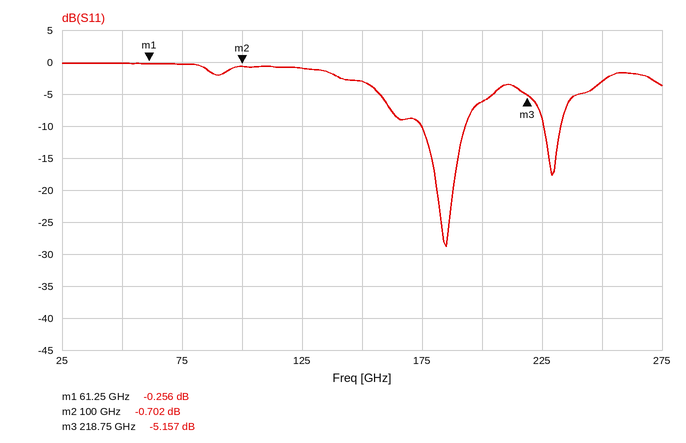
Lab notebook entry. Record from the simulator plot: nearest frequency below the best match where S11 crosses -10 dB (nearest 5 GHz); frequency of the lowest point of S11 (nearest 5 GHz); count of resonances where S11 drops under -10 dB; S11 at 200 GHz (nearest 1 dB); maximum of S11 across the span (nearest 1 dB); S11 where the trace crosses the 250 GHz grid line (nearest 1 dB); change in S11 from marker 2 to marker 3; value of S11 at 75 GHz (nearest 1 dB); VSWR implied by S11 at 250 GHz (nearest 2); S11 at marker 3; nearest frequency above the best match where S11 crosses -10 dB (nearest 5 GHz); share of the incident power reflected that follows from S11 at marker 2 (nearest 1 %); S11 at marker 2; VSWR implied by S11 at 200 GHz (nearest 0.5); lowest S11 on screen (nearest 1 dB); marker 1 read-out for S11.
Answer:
175 GHz
185 GHz
2
-6 dB
0 dB
-3 dB
-4.455 dB
0 dB
6
-5.157 dB
195 GHz
85 %
-0.702 dB
3.0
-29 dB
-0.256 dB
